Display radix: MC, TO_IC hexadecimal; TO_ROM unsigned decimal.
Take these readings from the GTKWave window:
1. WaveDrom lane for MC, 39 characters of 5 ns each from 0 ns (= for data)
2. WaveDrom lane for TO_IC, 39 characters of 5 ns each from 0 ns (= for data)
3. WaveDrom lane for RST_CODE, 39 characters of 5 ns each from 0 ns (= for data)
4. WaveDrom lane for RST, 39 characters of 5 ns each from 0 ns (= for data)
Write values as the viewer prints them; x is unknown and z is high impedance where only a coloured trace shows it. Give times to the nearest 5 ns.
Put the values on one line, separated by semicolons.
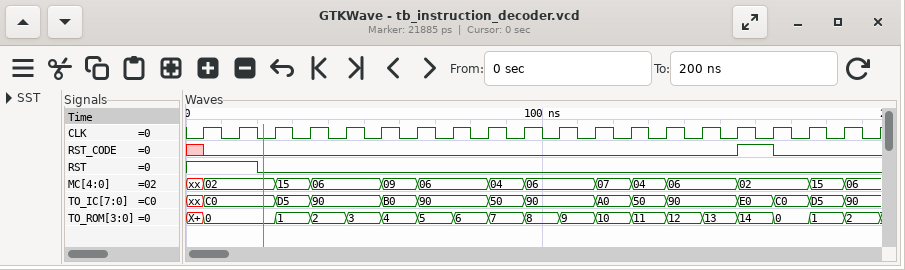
{name: 'MC', wave: 'x=...=.=...=.=...=.=...=.=.=...=...=.=.', data: '02 15 06 09 06 04 06 07 04 06 02 15 06'}; {name: 'TO_IC', wave: 'x=...=.=...=.=...=.=...=.=.=...=.=.=.=.', data: 'C0 D5 90 B0 90 50 90 A0 50 90 E0 C0 D5 90'}; {name: 'RST_CODE', wave: 'x0.............................1.0.....'}; {name: 'RST', wave: '1...0..................................'}
